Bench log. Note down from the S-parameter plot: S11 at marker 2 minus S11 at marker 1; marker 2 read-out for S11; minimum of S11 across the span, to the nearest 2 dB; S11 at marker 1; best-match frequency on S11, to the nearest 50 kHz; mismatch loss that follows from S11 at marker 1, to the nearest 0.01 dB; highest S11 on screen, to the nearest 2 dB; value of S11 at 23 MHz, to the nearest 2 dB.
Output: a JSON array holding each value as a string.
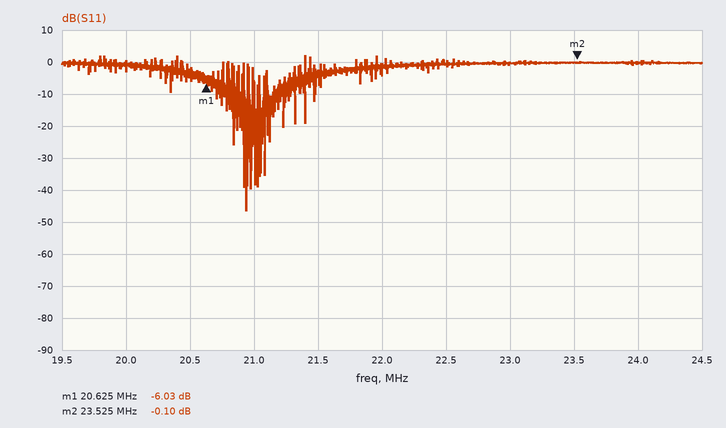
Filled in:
["5.93 dB", "-0.10 dB", "-46 dB", "-6.03 dB", "20.95 MHz", "1.25 dB", "2 dB", "0 dB"]
